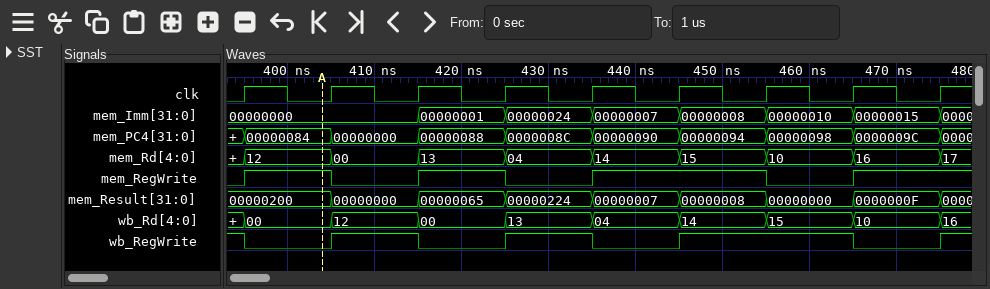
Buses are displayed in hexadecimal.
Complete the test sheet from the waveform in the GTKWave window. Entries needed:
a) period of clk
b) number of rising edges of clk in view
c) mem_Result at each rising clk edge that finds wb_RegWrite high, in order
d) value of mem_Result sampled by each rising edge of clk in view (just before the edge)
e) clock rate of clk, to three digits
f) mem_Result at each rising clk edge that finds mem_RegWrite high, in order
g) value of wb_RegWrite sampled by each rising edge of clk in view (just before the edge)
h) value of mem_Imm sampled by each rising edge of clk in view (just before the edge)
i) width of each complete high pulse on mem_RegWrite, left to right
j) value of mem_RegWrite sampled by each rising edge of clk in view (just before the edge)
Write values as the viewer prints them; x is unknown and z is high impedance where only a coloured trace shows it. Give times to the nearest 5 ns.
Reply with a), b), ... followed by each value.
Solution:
a) 10 ns
b) 9
c) 00000200, 00000000, 00000224, 00000008, 00000000
d) 00000200, 00000200, 00000000, 00000065, 00000224, 00000007, 00000008, 00000000, 0000000F
e) 100 MHz
f) 00000200, 00000065, 00000007, 00000008, 0000000F
g) 1 0 1 0 1 0 1 1 0
h) 00000000, 00000000, 00000000, 00000001, 00000024, 00000007, 00000008, 00000010, 00000015
i) 10 ns, 10 ns, 20 ns
j) 0 1 0 1 0 1 1 0 1
